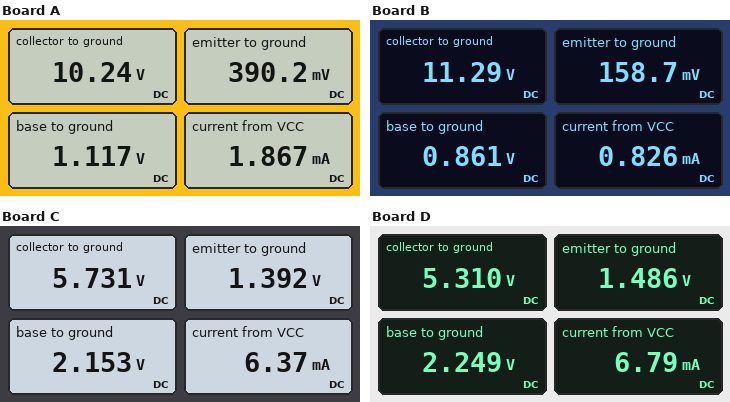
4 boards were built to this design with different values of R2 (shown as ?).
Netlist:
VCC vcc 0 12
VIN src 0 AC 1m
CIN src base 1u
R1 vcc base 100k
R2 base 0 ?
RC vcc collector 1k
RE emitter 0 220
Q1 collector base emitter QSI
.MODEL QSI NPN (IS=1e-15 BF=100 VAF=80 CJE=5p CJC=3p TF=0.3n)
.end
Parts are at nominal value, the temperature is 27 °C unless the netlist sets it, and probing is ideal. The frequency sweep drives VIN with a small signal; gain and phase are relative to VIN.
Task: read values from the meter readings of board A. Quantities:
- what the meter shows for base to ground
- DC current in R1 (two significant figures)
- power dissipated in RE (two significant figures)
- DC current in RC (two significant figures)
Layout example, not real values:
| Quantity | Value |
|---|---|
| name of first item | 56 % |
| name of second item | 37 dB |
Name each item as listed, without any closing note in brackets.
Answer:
| Quantity | Value |
|---|---|
| what the meter shows for base to ground | 1.117 V |
| DC current in R1 | 110 µA |
| power dissipated in RE | 690 µW |
| DC current in RC | 1.8 mA |
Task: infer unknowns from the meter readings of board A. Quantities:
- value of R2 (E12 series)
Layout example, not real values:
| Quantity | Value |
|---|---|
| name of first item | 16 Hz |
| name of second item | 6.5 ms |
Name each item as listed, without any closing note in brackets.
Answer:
| Quantity | Value |
|---|---|
| value of R2 | 12 kΩ |
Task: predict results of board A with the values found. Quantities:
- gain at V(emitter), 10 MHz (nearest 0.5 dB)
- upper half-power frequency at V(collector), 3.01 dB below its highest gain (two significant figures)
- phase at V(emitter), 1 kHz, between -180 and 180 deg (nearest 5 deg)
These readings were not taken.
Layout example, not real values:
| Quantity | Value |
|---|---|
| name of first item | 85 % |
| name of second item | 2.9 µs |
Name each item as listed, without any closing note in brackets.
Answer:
| Quantity | Value |
|---|---|
| gain at V(emitter), 10 MHz | -0.5 dB |
| upper half-power frequency at V(collector), 3.01 dB below its highest gain | 140 MHz |
| phase at V(emitter), 1 kHz, between -180 and 180 deg | 0 deg |
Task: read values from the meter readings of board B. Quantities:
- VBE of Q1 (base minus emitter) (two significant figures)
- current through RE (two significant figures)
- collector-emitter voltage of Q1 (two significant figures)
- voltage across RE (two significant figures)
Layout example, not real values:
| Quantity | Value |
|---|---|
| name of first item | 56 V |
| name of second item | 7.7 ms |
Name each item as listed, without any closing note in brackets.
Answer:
| Quantity | Value |
|---|---|
| VBE of Q1 (base minus emitter) | 700 mV |
| current through RE | 720 µA |
| collector-emitter voltage of Q1 | 11 V |
| voltage across RE | 160 mV |
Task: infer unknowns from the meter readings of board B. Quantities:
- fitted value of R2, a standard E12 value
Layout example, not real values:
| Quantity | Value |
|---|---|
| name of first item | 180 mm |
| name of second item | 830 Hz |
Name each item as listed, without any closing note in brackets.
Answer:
| Quantity | Value |
|---|---|
| fitted value of R2, a standard E12 value | 8.2 kΩ |
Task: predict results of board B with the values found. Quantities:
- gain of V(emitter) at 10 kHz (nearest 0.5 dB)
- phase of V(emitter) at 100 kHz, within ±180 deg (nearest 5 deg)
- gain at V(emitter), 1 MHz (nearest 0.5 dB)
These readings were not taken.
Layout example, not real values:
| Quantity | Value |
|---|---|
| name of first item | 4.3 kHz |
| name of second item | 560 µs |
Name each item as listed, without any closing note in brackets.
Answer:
| Quantity | Value |
|---|---|
| gain of V(emitter) at 10 kHz | -1.5 dB |
| phase of V(emitter) at 100 kHz, within ±180 deg | 0 deg |
| gain at V(emitter), 1 MHz | -1.5 dB |
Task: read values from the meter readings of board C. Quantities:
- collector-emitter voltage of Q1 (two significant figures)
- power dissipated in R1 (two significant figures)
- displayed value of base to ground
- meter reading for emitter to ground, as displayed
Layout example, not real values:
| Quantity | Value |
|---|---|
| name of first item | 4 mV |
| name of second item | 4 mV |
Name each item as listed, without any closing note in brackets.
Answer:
| Quantity | Value |
|---|---|
| collector-emitter voltage of Q1 | 4.3 V |
| power dissipated in R1 | 970 µW |
| displayed value of base to ground | 2.153 V |
| meter reading for emitter to ground, as displayed | 1.392 V |
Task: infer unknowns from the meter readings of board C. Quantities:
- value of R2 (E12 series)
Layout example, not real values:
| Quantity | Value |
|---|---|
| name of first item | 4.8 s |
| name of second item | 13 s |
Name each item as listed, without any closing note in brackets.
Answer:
| Quantity | Value |
|---|---|
| value of R2 | 56 kΩ |
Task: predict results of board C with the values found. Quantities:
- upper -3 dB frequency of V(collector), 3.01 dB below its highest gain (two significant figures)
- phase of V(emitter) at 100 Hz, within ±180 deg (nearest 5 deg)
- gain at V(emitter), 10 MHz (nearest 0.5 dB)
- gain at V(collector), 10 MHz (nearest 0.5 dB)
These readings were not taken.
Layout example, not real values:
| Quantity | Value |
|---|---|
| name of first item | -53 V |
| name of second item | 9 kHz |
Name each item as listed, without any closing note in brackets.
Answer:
| Quantity | Value |
|---|---|
| upper -3 dB frequency of V(collector), 3.01 dB below its highest gain | 110 MHz |
| phase of V(emitter) at 100 Hz, within ±180 deg | 5 deg |
| gain at V(emitter), 10 MHz | 0 dB |
| gain at V(collector), 10 MHz | 13.0 dB |
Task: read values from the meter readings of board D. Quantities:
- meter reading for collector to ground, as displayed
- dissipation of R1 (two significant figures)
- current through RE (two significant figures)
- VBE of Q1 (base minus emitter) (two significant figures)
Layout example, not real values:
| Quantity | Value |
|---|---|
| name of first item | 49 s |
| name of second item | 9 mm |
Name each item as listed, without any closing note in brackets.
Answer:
| Quantity | Value |
|---|---|
| meter reading for collector to ground, as displayed | 5.310 V |
| dissipation of R1 | 950 µW |
| current through RE | 6.8 mA |
| VBE of Q1 (base minus emitter) | 760 mV |
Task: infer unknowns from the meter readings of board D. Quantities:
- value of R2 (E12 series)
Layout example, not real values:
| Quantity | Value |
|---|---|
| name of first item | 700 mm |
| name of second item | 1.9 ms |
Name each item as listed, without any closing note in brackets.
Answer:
| Quantity | Value |
|---|---|
| value of R2 | 68 kΩ |
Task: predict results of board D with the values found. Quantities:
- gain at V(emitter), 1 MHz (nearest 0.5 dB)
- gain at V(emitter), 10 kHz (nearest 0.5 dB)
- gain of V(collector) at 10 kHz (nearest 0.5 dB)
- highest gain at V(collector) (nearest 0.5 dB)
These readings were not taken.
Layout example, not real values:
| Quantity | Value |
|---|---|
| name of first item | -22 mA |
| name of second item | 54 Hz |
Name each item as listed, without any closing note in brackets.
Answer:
| Quantity | Value |
|---|---|
| gain at V(emitter), 1 MHz | 0 dB |
| gain at V(emitter), 10 kHz | 0 dB |
| gain of V(collector) at 10 kHz | 13.0 dB |
| highest gain at V(collector) | 13.0 dB |
